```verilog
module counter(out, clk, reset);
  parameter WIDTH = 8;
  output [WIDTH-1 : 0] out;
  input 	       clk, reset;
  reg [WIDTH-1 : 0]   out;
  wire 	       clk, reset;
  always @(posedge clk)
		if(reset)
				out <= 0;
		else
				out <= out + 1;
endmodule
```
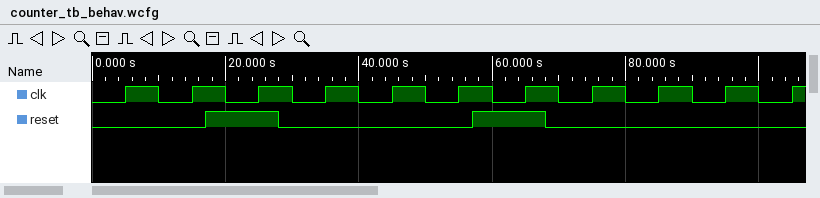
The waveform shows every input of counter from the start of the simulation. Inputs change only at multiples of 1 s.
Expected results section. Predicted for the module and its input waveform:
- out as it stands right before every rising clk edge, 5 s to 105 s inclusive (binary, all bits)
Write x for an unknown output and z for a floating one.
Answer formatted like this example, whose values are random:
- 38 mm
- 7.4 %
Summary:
- x, x, x, 00000000, 00000001, 00000010, 00000011, 00000000, 00000001, 00000010, 00000011
